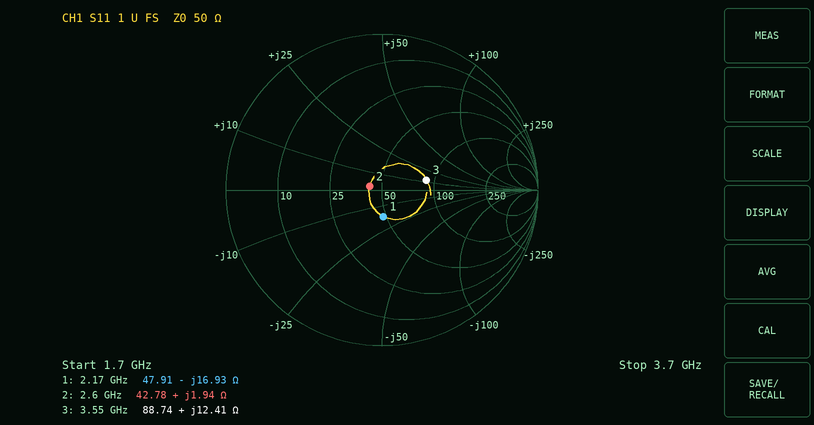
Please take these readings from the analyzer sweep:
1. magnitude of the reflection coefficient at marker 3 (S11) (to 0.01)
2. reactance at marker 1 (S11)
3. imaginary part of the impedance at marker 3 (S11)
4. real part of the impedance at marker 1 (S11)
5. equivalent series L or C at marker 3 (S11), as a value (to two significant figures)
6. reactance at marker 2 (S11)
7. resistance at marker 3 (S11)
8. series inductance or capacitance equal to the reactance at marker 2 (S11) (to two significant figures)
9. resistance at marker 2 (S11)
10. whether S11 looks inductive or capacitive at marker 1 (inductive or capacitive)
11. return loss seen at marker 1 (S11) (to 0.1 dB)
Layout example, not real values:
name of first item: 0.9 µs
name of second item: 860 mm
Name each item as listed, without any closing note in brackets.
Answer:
magnitude of the reflection coefficient at marker 3 (S11): 0.29
reactance at marker 1: -16.93 Ω
imaginary part of the impedance at marker 3: +12.41 Ω
real part of the impedance at marker 1: 47.91 Ω
equivalent series L or C at marker 3 (S11), as a value: 560 pH
reactance at marker 2: +1.94 Ω
resistance at marker 3: 88.74 Ω
series inductance or capacitance equal to the reactance at marker 2 (S11): 120 pH
resistance at marker 2: 42.78 Ω
whether S11 looks inductive or capacitive at marker 1: capacitive
return loss seen at marker 1 (S11): 15.3 dB
